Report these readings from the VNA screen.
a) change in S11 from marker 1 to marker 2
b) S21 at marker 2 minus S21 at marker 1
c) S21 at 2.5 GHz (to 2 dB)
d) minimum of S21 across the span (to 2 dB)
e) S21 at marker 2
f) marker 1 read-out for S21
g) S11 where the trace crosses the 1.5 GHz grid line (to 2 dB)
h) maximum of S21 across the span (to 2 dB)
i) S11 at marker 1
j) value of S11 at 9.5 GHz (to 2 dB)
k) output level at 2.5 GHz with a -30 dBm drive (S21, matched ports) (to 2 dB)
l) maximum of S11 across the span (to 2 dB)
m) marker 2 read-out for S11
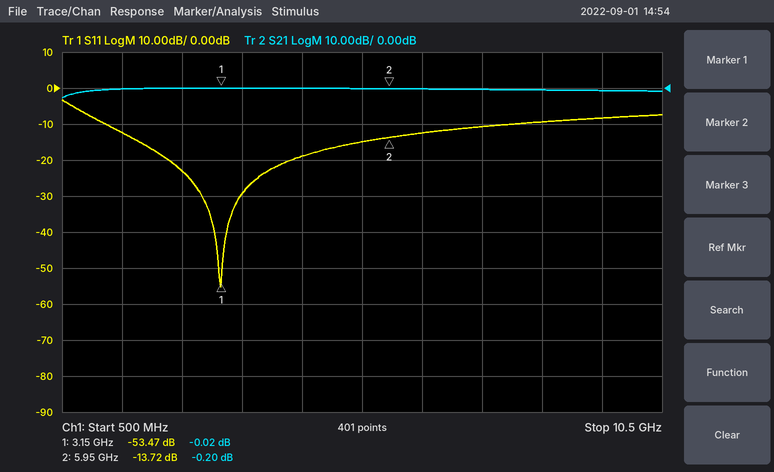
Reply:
39.75 dB
-0.18 dB
0 dB
-2 dB
-0.20 dB
-0.02 dB
-12 dB
0 dB
-53.47 dB
-8 dB
-30 dBm
-4 dB
-13.72 dB
